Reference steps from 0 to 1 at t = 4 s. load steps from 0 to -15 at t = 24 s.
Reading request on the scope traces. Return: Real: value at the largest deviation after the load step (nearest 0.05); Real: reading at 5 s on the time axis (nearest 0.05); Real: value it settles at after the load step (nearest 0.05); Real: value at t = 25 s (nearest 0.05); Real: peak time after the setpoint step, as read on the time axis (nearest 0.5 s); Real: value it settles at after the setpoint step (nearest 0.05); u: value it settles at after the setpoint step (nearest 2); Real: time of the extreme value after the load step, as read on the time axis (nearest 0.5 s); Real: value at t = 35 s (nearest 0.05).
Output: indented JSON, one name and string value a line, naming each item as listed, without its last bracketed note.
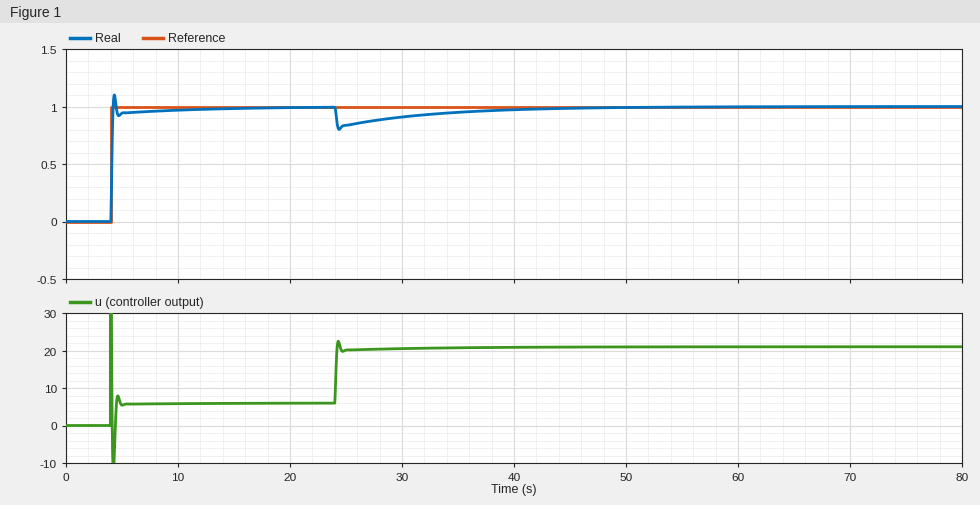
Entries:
{
  "Real: value at the largest deviation after the load step": "0.80",
  "Real: reading at 5 s on the time axis": "0.95",
  "Real: value it settles at after the load step": "1.00",
  "Real: value at t = 25 s": "0.85",
  "Real: peak time after the setpoint step, as read on the time axis": "4.5 s",
  "Real: value it settles at after the setpoint step": "1.00",
  "u: value it settles at after the setpoint step": "6",
  "Real: time of the extreme value after the load step, as read on the time axis": "24.5 s",
  "Real: value at t = 35 s": "0.95"
}
